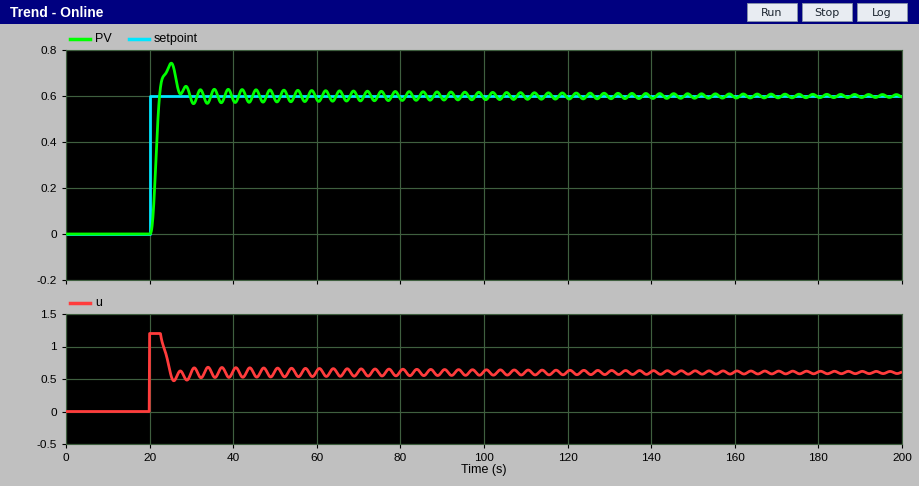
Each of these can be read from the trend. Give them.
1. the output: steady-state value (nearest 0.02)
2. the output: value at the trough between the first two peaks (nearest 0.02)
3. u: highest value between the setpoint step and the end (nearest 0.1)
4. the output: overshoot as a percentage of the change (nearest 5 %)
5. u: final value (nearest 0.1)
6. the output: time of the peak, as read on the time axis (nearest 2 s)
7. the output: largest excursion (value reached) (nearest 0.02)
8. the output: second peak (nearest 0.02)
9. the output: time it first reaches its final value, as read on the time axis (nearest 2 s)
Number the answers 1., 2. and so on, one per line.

1. 0.60
2. 0.56
3. 1.2
4. 25 %
5. 0.6
6. 26 s
7. 0.74
8. 0.62
9. 22 s
